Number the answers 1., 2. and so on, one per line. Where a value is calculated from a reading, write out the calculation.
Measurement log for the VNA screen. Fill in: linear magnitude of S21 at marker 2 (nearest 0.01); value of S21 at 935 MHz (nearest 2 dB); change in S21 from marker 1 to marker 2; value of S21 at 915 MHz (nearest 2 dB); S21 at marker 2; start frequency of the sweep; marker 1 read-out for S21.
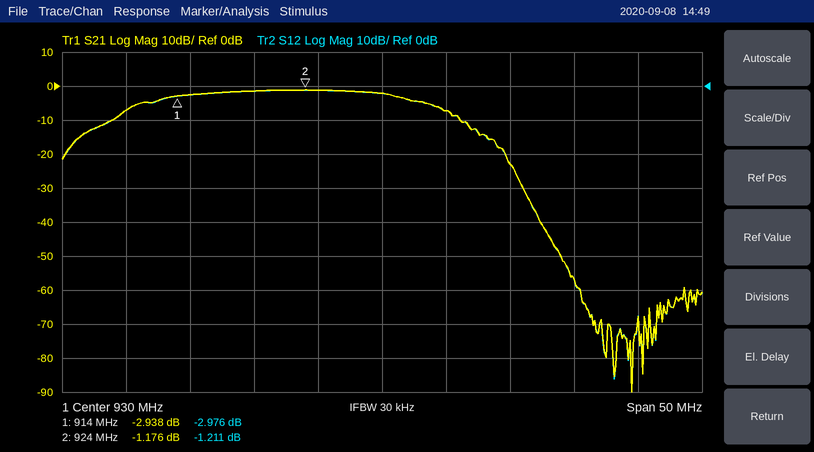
1. 10^(-1.176/20) ≈ 0.87
2. -8 dB
3. -1.176 − (-2.938) = 1.762 dB
4. -2 dB
5. -1.176 dB
6. 905 MHz
7. -2.938 dB
